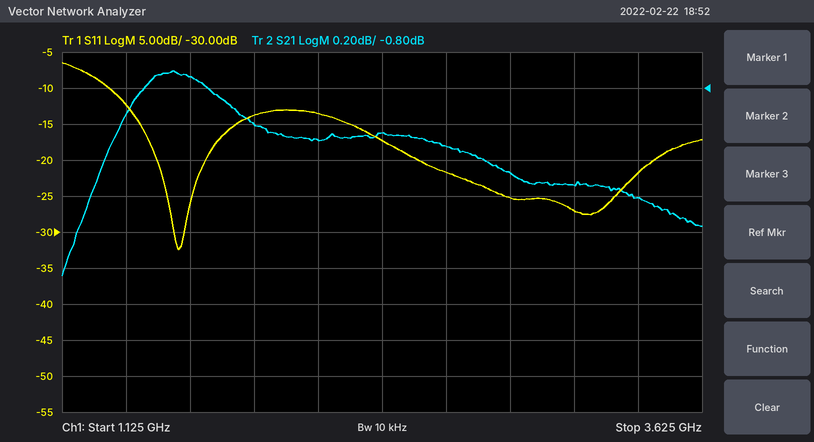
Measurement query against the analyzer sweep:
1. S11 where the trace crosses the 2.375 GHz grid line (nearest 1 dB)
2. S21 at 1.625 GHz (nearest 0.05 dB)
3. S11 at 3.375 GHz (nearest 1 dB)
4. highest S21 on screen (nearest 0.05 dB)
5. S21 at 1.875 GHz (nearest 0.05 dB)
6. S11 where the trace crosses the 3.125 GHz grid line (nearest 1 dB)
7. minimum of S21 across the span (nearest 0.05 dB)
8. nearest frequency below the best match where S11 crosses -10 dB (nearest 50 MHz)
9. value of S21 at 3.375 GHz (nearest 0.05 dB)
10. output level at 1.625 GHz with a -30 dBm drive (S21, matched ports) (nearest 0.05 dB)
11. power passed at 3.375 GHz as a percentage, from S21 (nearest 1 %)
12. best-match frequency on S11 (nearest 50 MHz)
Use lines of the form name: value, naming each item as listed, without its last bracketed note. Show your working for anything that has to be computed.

S11 where the trace crosses the 2.375 GHz grid line: -17 dB
S21 at 1.625 GHz: -0.75 dB
S11 at 3.375 GHz: -22 dB
highest S21 on screen: -0.70 dB
S21 at 1.875 GHz: -1.00 dB
S11 where the trace crosses the 3.125 GHz grid line: -27 dB
minimum of S21 across the span: -1.85 dB
nearest frequency below the best match where S11 crosses -10 dB: 1.30 GHz
value of S21 at 3.375 GHz: -1.40 dB
output level at 1.625 GHz with a -30 dBm drive (S21, matched ports): -30 dBm + (-0.75 dB) = -30.75 dBm
power passed at 3.375 GHz as a percentage, from S21: 10^(-1.4/10) ≈ 72 %
best-match frequency on S11: 1.60 GHz
